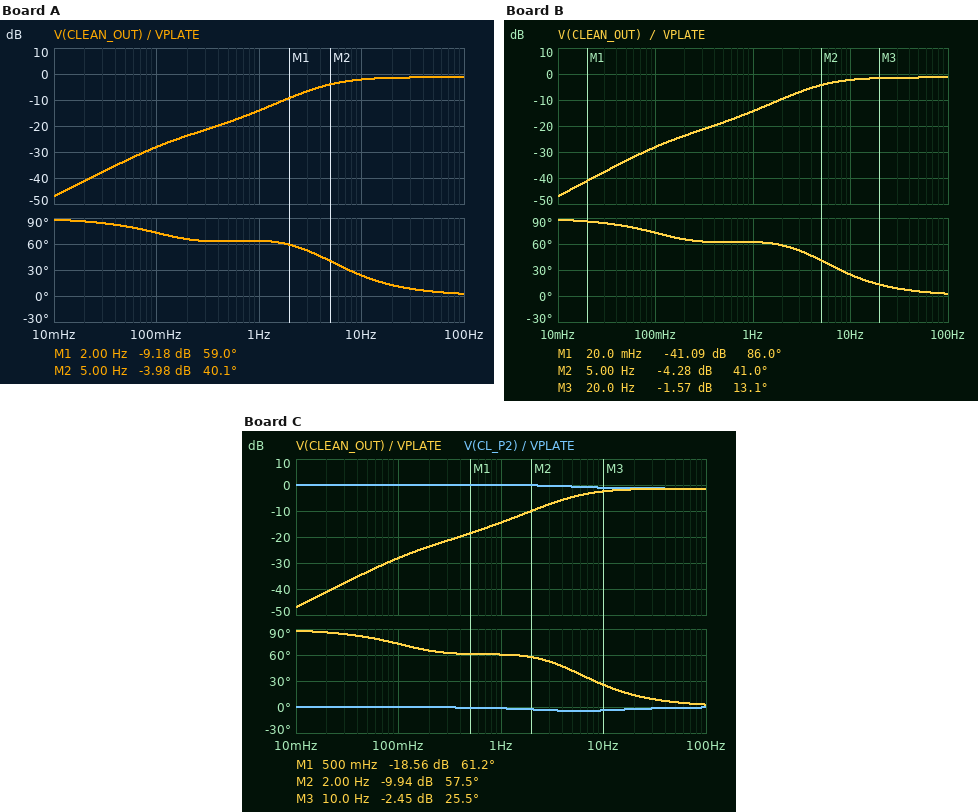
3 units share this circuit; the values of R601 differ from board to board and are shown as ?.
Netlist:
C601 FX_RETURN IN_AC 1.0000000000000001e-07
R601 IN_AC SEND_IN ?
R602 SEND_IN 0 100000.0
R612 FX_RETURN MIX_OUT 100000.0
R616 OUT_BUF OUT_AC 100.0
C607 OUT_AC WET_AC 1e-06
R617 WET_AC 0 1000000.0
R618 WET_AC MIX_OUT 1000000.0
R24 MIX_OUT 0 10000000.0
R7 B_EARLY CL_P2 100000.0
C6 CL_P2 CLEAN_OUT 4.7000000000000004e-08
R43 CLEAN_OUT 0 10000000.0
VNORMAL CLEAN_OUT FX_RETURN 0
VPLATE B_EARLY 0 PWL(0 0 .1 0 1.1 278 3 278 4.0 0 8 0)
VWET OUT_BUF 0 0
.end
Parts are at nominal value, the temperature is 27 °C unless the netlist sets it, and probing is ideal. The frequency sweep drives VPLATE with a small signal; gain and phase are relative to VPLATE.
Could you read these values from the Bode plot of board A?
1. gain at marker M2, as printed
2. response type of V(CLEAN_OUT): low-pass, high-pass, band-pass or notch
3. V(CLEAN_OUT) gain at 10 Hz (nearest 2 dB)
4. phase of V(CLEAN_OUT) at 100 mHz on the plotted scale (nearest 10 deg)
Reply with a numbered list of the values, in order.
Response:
1. -3.98 dB
2. high-pass
3. -2 dB
4. 70 deg
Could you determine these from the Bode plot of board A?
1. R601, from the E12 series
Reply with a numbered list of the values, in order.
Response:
1. 2.2 MΩ
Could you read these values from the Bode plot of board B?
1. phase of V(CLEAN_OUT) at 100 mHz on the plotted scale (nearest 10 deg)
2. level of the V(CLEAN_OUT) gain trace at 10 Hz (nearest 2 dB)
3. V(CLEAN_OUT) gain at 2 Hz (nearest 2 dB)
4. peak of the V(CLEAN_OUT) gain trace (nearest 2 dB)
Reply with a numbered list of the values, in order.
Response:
1. 70 deg
2. -2 dB
3. -10 dB
4. -2 dB
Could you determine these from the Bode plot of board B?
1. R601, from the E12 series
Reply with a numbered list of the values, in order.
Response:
1. 1.8 MΩ
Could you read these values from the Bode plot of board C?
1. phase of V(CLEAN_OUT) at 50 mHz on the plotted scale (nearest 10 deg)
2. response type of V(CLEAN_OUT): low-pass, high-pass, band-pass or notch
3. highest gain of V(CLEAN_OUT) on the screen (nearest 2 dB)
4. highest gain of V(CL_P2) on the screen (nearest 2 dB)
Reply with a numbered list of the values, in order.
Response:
1. 80 deg
2. high-pass
3. -2 dB
4. 0 dB
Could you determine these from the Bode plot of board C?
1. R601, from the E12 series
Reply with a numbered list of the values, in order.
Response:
1. 1.5 MΩ
